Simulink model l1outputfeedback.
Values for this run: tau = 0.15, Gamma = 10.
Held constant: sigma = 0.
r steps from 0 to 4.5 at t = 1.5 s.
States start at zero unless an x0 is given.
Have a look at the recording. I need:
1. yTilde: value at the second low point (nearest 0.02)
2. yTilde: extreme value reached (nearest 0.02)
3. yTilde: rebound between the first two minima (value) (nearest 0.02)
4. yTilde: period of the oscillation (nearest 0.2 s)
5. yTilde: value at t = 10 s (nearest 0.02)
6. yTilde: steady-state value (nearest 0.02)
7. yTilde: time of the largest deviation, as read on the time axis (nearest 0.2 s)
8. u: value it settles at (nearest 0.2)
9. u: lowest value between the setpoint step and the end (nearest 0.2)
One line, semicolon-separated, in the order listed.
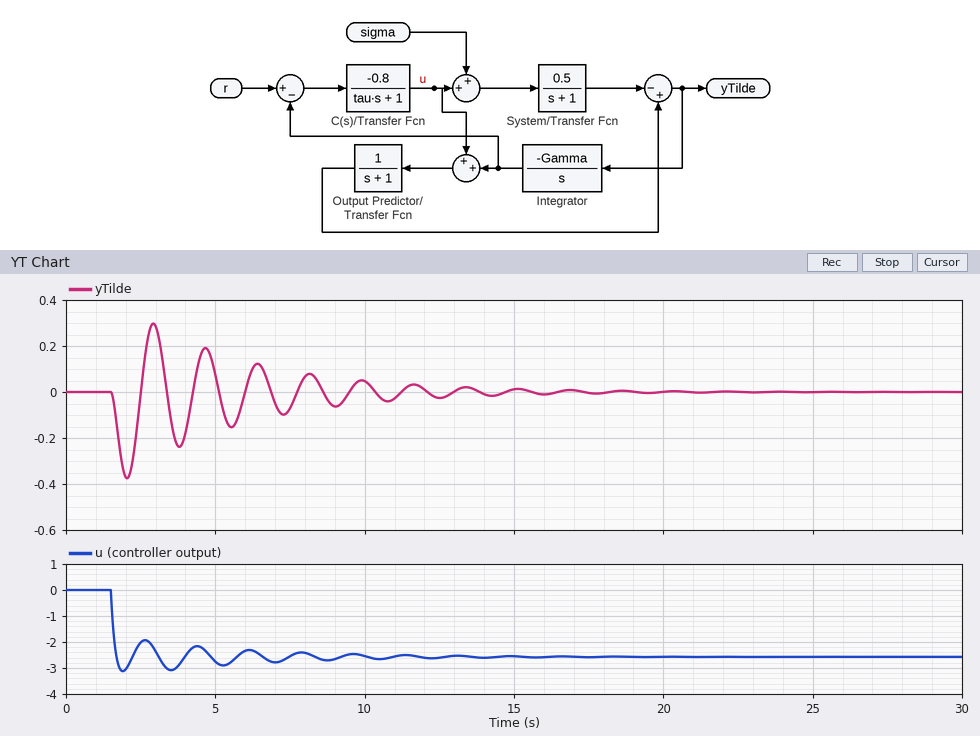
-0.24; -0.38; 0.30; 1.8 s; 0.04; 0.00; 2.0 s; -2.6; -3.2
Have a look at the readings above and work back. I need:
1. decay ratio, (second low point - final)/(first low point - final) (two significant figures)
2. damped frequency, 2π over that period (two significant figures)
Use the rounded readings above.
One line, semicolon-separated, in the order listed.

0.63; 3.5 rad/s
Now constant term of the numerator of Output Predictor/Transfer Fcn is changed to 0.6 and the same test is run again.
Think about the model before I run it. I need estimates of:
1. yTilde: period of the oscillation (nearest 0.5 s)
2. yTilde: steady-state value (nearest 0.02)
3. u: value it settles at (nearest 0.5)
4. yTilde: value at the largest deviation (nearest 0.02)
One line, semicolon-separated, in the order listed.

2.5 s; 0.00; -3.0; -0.10
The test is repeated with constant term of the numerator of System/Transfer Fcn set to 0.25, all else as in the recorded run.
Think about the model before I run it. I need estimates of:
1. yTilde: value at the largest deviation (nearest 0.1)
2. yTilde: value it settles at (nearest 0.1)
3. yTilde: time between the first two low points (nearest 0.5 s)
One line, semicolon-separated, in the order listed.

-0.5; 0.0; 1.5 s
